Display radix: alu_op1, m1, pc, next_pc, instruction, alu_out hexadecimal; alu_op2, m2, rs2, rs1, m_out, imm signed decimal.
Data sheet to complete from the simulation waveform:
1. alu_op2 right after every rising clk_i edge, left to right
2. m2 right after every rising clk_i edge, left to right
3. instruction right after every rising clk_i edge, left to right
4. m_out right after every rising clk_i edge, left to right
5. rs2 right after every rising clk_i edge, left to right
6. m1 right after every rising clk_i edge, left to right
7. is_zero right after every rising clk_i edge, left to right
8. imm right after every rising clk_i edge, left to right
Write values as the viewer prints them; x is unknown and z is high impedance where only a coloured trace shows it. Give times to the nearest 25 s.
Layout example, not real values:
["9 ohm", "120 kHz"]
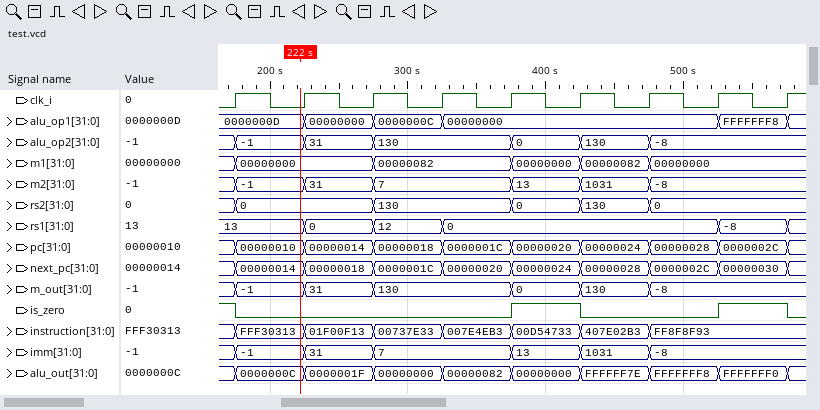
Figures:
["-1, 31, 130, 130, 0, 130, -8, -8, -8", "-1, 31, 7, 7, 13, 1031, -8, -8, -8", "FFF30313, 01F00F13, 00737E33, 007E4EB3, 00D54733, 407E02B3, FF8F8F93, FF8F8F93, FF8F8F93", "-1, 31, 130, 130, 0, 130, -8, -8, -8", "0, 0, 130, 130, 0, 130, 0, 0, 0", "00000000, 00000000, 00000082, 00000082, 00000000, 00000082, 00000000, 00000000, 00000000", "0 0 0 0 1 0 0 1 0", "-1, 31, 7, 7, 13, 1031, -8, -8, -8"]
